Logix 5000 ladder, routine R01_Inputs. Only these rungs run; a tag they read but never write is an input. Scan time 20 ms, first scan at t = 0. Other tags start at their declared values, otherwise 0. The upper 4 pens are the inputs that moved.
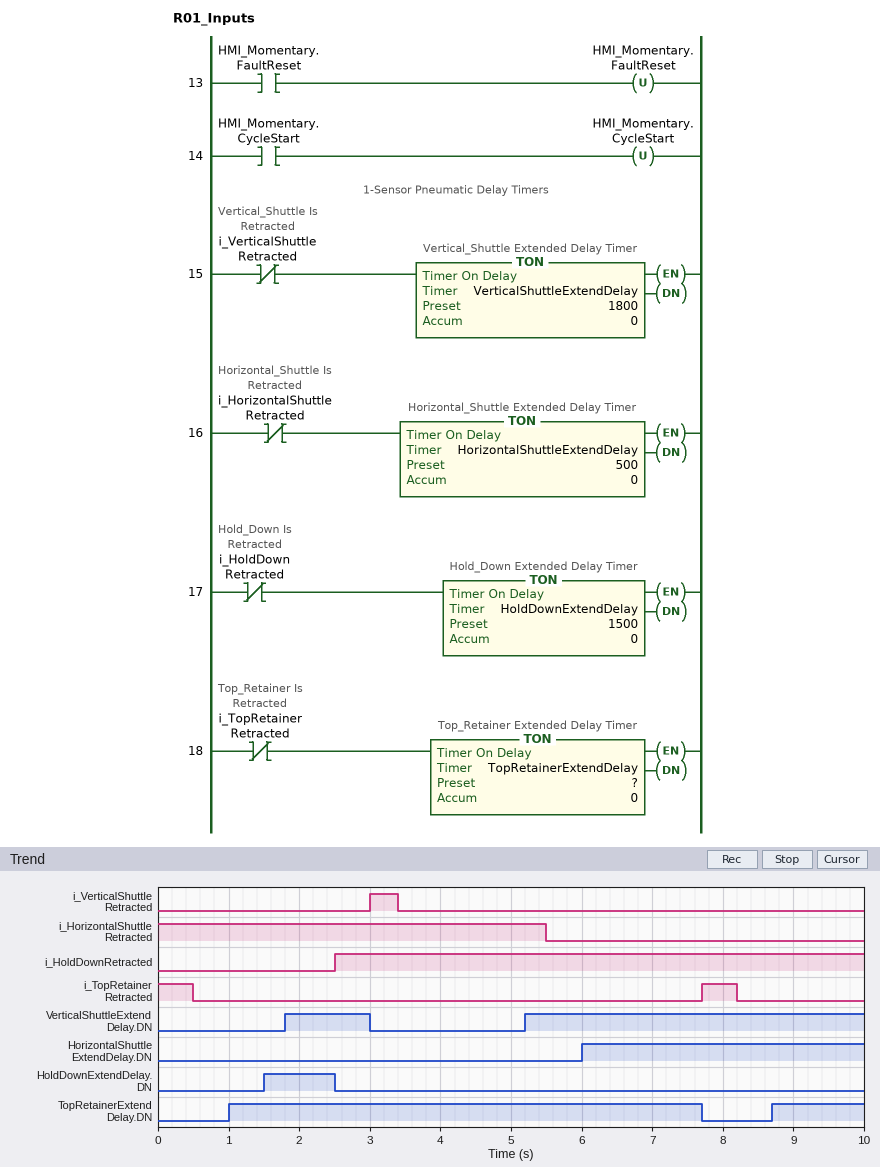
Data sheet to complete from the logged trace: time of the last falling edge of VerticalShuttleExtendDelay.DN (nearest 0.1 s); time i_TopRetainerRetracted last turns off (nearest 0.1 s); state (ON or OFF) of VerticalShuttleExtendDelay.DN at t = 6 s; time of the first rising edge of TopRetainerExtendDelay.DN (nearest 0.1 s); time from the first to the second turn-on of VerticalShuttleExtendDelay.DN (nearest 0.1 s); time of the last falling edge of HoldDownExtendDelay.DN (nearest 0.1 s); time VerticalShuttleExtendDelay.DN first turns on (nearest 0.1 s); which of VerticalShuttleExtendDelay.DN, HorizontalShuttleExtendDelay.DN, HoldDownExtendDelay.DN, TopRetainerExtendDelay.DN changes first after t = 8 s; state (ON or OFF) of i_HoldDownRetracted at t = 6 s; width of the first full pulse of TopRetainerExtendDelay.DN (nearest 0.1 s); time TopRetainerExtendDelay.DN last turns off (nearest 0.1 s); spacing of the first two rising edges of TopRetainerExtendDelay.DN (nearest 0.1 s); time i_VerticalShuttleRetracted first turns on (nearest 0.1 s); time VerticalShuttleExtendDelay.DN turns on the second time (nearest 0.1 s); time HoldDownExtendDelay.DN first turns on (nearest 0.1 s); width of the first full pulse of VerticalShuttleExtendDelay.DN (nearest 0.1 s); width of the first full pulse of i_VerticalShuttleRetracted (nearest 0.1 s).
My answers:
3.0 s
8.2 s
ON
1.0 s
3.4 s
2.5 s
1.8 s
TopRetainerExtendDelay.DN
ON
6.7 s
7.7 s
7.7 s
3.0 s
5.2 s
1.5 s
1.2 s
0.4 s
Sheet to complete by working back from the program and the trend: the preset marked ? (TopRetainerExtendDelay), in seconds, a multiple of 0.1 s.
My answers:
0.5 s
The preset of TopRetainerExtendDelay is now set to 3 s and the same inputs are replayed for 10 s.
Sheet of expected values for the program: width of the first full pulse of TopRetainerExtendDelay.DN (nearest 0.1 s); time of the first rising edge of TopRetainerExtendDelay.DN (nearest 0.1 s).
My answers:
4.2 s
3.5 s
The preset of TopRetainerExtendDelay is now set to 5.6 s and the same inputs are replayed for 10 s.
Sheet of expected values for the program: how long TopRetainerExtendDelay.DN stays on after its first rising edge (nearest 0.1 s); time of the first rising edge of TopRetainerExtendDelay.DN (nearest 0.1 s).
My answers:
1.6 s
6.1 s
